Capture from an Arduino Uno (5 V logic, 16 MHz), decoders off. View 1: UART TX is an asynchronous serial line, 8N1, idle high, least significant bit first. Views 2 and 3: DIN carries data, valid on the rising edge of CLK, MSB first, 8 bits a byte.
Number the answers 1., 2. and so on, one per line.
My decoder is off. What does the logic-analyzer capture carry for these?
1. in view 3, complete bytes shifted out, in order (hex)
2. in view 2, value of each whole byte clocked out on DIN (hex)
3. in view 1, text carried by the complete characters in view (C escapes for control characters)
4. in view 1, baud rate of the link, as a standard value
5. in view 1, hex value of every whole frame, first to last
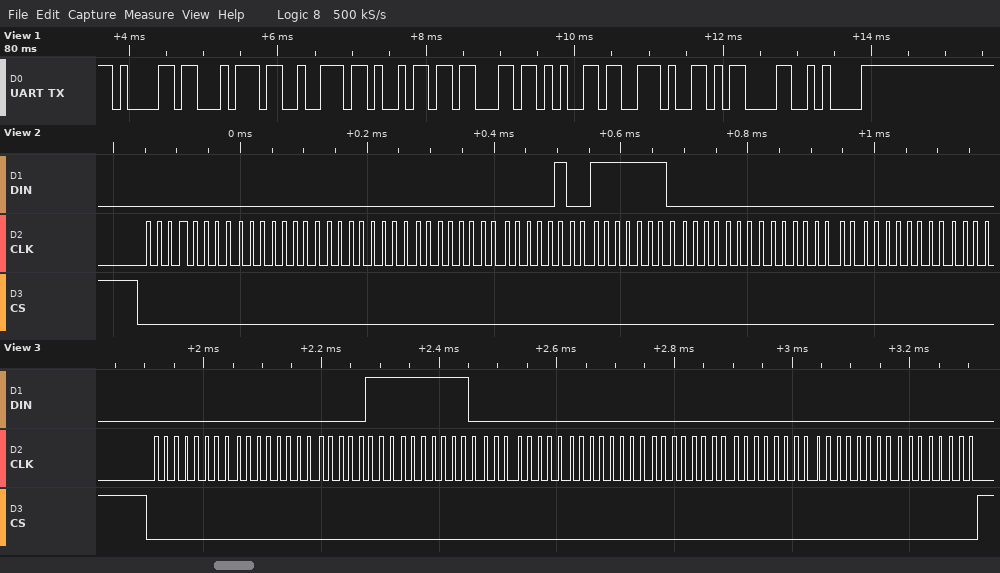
1. 00 00 07 FE 00 00 00 00 00 00
2. 00 00 00 00 04 FE 00 00 00
3. "atrice.\r\n"
4. 9600 baud
5. 0x61 0x74 0x72 0x69 0x63 0x65 0x2E 0x0D 0x0A
